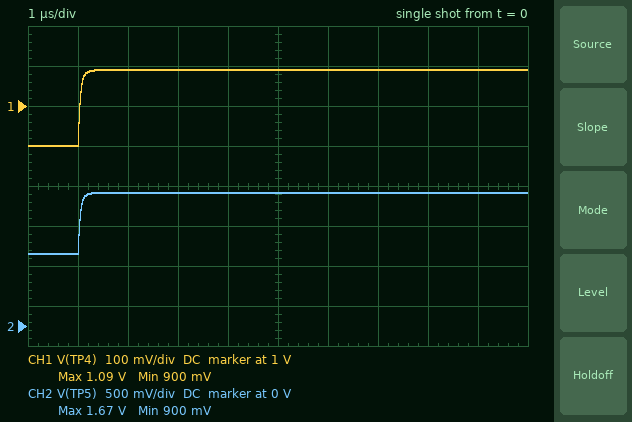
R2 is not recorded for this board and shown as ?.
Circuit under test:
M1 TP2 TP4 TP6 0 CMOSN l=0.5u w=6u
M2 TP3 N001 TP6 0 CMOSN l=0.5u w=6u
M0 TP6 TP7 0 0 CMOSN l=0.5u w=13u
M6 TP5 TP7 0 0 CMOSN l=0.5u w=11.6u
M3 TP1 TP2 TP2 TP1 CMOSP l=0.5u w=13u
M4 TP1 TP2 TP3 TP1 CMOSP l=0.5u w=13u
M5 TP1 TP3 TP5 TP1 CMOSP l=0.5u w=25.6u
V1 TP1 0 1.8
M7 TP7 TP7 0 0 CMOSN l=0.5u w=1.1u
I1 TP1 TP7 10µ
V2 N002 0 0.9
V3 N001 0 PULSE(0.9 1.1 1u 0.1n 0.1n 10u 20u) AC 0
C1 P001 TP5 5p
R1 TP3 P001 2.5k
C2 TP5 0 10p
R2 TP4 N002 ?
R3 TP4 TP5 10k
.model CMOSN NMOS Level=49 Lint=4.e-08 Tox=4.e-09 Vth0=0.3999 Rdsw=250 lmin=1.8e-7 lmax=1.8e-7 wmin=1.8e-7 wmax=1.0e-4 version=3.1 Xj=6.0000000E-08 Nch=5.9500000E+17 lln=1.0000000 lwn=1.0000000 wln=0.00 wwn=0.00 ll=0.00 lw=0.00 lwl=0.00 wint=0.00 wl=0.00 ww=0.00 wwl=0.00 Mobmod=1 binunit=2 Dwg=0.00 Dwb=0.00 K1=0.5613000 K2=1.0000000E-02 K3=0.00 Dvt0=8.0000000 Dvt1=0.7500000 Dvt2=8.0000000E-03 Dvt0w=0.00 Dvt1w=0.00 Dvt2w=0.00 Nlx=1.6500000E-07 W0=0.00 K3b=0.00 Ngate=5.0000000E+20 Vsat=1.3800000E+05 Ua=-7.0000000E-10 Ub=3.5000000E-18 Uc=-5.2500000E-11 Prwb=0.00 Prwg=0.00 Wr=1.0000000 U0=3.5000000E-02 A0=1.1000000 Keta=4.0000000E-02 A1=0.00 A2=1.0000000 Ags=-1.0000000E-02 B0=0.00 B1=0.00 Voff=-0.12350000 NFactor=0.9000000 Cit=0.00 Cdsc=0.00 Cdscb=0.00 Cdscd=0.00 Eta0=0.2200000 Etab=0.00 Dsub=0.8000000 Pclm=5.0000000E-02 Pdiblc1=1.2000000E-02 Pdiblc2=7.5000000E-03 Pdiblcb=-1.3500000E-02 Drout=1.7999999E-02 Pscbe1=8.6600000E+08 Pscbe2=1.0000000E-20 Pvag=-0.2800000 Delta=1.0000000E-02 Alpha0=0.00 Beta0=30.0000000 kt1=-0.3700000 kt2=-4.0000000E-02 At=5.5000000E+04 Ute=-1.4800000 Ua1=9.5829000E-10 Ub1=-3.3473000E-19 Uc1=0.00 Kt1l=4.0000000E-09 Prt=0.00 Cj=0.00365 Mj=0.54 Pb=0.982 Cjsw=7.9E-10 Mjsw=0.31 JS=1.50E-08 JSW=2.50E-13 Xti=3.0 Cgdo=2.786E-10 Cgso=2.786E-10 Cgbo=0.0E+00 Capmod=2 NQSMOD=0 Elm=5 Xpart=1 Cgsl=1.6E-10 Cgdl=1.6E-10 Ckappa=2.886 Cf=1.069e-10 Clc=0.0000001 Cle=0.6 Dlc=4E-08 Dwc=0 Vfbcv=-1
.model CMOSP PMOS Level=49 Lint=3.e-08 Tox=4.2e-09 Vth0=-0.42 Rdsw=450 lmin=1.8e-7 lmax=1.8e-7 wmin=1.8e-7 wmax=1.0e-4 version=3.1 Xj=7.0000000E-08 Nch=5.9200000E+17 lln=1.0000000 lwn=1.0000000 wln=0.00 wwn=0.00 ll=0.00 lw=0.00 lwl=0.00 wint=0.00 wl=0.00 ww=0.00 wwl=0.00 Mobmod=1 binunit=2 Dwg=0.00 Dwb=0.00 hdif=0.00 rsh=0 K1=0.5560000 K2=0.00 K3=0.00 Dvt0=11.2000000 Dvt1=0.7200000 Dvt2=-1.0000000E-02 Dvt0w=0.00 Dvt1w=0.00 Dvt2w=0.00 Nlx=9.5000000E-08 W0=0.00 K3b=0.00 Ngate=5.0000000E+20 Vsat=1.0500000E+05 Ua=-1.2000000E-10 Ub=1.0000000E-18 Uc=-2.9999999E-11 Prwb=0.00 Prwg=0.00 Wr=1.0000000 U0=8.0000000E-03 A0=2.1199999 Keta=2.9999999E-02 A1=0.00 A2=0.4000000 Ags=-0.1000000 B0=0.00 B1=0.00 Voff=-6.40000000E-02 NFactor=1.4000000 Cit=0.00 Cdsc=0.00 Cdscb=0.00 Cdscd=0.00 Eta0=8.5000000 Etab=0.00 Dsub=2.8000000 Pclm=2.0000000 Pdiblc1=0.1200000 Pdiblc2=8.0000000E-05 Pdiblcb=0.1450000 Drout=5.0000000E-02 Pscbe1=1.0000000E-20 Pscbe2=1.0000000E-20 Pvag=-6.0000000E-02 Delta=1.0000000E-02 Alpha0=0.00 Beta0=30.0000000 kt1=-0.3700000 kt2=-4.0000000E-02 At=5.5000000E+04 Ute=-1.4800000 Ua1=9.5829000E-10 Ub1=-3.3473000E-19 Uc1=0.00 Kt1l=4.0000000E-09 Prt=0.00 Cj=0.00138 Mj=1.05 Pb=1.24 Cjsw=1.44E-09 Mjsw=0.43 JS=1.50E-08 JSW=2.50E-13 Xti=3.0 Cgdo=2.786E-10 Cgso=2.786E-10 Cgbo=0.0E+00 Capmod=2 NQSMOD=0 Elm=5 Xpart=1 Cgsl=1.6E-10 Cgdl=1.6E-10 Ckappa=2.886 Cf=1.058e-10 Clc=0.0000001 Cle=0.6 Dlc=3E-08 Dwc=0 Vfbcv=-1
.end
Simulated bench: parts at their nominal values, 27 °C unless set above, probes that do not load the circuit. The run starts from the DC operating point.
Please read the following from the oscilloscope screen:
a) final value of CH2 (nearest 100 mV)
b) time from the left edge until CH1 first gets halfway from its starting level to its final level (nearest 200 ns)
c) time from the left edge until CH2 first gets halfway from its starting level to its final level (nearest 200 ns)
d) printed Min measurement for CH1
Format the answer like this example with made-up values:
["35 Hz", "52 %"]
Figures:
["1.7 V", "1.0 µs", "1.0 µs", "900 mV"]
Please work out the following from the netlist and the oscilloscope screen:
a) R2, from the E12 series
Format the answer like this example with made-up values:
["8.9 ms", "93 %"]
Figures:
["3.3 kΩ"]
